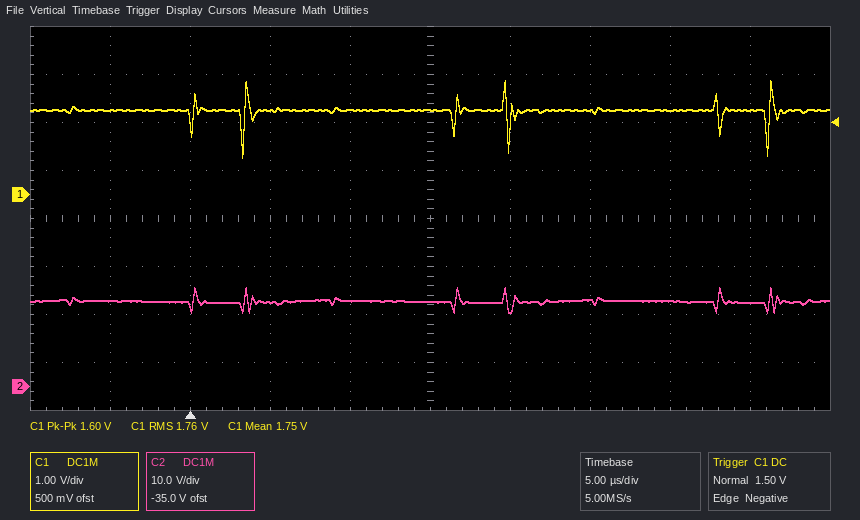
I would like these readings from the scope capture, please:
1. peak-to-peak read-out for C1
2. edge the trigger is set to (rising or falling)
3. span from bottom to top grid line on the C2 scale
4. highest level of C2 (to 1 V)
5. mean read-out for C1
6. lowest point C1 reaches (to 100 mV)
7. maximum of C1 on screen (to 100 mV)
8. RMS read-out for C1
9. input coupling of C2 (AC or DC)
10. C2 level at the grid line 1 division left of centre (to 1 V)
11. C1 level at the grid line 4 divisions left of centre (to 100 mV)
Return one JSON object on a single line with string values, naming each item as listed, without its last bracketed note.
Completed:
{"peak-to-peak read-out for C1": "1.60 V", "edge the trigger is set to": "falling", "span from bottom to top grid line on the C2 scale": "80 V", "highest level of C2": "21 V", "mean read-out for C1": "1.75 V", "lowest point C1 reaches": "800 mV", "maximum of C1 on screen": "2.4 V", "RMS read-out for C1": "1.76 V", "input coupling of C2": "DC", "C2 level at the grid line 1 division left of centre": "18 V", "C1 level at the grid line 4 divisions left of centre": "1.8 V"}
